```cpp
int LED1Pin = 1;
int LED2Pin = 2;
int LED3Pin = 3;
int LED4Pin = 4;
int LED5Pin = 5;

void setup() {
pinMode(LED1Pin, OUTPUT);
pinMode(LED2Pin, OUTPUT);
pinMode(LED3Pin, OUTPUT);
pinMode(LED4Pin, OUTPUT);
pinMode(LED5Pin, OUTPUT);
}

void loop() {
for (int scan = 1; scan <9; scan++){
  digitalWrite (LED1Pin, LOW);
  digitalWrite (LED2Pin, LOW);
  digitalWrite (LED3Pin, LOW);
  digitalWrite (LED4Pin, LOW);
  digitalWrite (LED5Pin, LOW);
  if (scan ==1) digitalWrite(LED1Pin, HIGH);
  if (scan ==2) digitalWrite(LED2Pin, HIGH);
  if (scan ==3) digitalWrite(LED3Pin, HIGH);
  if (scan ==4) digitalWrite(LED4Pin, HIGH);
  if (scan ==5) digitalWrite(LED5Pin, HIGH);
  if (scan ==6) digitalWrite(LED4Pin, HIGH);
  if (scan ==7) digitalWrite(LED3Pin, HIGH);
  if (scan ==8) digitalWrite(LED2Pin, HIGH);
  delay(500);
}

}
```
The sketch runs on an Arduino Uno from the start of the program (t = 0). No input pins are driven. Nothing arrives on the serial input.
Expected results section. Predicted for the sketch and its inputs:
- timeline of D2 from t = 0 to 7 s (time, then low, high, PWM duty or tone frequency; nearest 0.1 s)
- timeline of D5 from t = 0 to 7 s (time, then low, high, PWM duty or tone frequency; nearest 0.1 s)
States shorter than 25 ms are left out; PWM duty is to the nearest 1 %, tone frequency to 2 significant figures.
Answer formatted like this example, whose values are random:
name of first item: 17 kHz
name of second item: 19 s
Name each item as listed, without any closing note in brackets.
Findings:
timeline of D2 from t = 0 to 7 s: 0 s low; 0.5 s high; 1 s low; 3.5 s high; 4 s low; 4.5 s high; 5 s low
timeline of D5 from t = 0 to 7 s: 0 s low; 2 s high; 2.5 s low; 6 s high; 6.5 s low
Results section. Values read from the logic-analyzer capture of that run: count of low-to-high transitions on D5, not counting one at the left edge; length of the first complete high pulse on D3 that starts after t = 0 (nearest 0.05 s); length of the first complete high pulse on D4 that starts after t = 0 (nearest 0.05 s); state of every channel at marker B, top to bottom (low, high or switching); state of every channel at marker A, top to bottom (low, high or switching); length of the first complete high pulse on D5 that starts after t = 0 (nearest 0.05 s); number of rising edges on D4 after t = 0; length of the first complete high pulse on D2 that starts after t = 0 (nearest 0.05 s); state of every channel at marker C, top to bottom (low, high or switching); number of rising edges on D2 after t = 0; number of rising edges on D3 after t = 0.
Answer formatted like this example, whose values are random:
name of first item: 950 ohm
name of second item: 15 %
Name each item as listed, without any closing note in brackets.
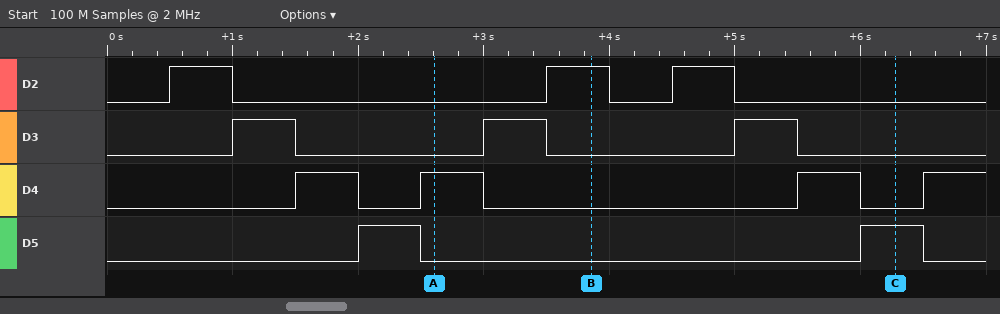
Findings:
count of low-to-high transitions on D5, not counting one at the left edge: 2
length of the first complete high pulse on D3 that starts after t = 0: 0.50 s
length of the first complete high pulse on D4 that starts after t = 0: 0.50 s
state of every channel at marker B, top to bottom: D2 high, D3 low, D4 low, D5 low
state of every channel at marker A, top to bottom: D2 low, D3 low, D4 high, D5 low
length of the first complete high pulse on D5 that starts after t = 0: 0.50 s
number of rising edges on D4 after t = 0: 4
length of the first complete high pulse on D2 that starts after t = 0: 0.50 s
state of every channel at marker C, top to bottom: D2 low, D3 low, D4 low, D5 high
number of rising edges on D2 after t = 0: 3
number of rising edges on D3 after t = 0: 3
